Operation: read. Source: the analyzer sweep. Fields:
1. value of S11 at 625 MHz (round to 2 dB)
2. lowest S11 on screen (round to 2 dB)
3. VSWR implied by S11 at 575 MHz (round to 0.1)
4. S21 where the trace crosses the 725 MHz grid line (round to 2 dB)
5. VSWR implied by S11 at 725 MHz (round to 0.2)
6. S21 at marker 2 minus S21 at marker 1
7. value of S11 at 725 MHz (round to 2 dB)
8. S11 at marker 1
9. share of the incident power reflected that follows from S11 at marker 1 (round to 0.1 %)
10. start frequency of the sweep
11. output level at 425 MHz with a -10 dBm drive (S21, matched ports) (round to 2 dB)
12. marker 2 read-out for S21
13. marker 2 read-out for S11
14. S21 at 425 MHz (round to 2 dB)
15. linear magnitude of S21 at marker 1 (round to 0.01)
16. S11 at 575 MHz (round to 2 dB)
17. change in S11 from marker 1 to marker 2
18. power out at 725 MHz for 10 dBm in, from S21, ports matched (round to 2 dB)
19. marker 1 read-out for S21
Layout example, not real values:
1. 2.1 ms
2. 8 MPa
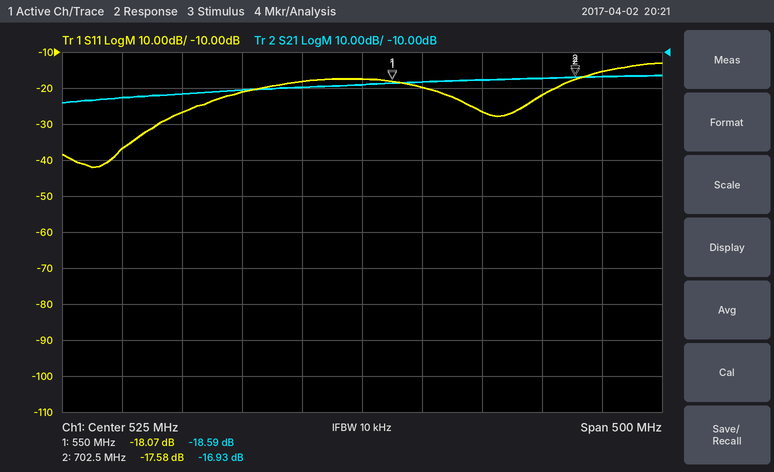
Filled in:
1. -26 dB
2. -42 dB
3. 1.2
4. -16 dB
5. 1.4
6. 1.66 dB
7. -16 dB
8. -18.07 dB
9. 1.6 %
10. 275 MHz
11. -30 dBm
12. -16.93 dB
13. -17.58 dB
14. -20 dB
15. 0.12
16. -20 dB
17. 0.49 dB
18. -6 dBm
19. -18.59 dB
